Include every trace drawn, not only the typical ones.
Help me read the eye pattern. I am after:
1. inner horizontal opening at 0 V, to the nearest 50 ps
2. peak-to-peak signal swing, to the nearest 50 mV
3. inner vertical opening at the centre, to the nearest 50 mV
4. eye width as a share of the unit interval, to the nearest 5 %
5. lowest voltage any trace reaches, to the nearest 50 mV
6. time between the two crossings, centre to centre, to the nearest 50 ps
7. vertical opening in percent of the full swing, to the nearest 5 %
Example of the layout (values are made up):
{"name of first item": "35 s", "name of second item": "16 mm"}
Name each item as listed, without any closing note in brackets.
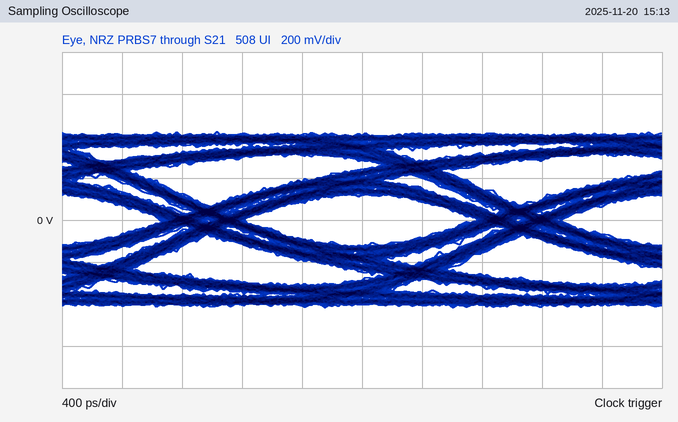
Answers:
{"inner horizontal opening at 0 V, to the nearest 50 ps": "1.55 ns", "peak-to-peak signal swing, to the nearest 50 mV": "850 mV", "inner vertical opening at the centre, to the nearest 50 mV": "250 mV", "eye width as a share of the unit interval, to the nearest 5 %": "75 %", "lowest voltage any trace reaches, to the nearest 50 mV": "-400 mV", "time between the two crossings, centre to centre, to the nearest 50 ps": "2.10 ns", "vertical opening in percent of the full swing, to the nearest 5 %": "30 %"}
